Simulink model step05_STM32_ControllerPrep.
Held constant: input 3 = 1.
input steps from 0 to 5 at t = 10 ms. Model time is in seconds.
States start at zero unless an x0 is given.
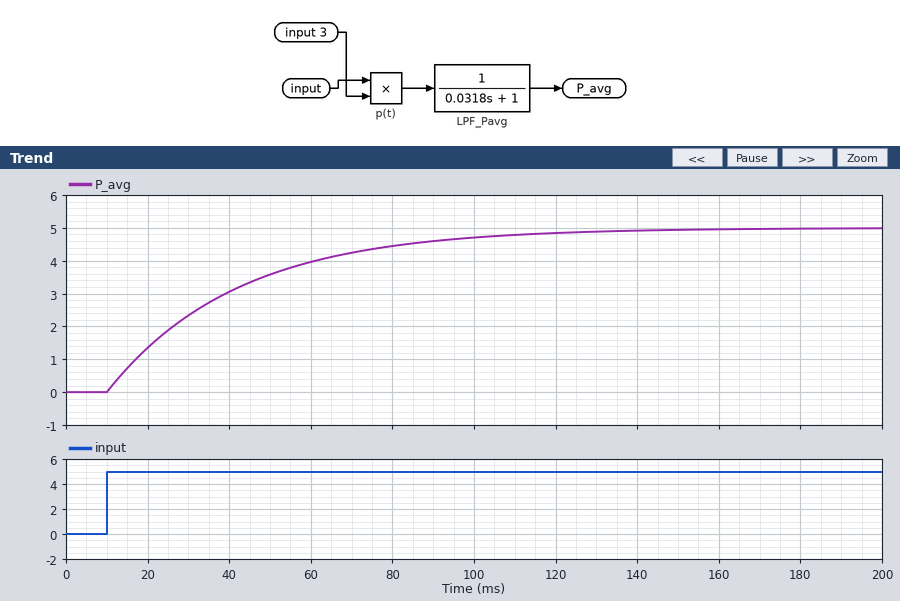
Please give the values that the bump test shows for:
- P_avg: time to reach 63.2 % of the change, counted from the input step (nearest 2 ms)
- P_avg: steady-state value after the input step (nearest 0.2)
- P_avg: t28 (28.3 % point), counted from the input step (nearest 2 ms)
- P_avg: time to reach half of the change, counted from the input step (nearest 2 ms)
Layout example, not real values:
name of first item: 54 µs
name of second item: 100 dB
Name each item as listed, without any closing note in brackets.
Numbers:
P_avg: time to reach 63.2 % of the change, counted from the input step: 32 ms
P_avg: steady-state value after the input step: 5.0
P_avg: t28 (28.3 % point), counted from the input step: 10 ms
P_avg: time to reach half of the change, counted from the input step: 22 ms
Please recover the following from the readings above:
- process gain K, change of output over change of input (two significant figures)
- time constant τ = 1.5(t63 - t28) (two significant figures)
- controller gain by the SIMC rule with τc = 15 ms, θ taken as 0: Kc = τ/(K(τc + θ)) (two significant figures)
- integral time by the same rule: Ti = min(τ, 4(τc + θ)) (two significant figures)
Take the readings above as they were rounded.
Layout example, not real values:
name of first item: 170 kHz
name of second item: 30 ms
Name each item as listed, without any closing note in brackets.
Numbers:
process gain K, change of output over change of input: 1.0
time constant τ = 1.5(t63 - t28): 33 ms
controller gain by the SIMC rule with τc = 15 ms, θ taken as 0: Kc = τ/(K(τc + θ)): 2.2
integral time by the same rule: Ti = min(τ, 4(τc + θ)): 33 ms
